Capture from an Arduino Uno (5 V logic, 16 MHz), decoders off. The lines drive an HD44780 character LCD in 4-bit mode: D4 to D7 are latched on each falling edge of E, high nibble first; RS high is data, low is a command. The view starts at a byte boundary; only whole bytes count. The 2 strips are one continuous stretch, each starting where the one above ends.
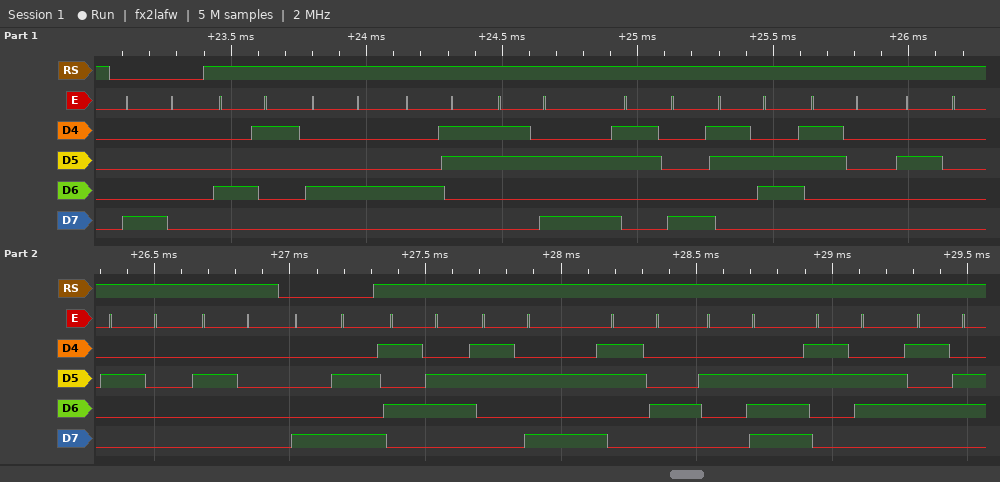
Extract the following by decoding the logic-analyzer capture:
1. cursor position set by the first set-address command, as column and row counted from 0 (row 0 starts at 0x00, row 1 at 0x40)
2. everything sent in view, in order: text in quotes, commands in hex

column 0, row 0
0x80 "ADC:860   " 0x8A "V:4.6V"
